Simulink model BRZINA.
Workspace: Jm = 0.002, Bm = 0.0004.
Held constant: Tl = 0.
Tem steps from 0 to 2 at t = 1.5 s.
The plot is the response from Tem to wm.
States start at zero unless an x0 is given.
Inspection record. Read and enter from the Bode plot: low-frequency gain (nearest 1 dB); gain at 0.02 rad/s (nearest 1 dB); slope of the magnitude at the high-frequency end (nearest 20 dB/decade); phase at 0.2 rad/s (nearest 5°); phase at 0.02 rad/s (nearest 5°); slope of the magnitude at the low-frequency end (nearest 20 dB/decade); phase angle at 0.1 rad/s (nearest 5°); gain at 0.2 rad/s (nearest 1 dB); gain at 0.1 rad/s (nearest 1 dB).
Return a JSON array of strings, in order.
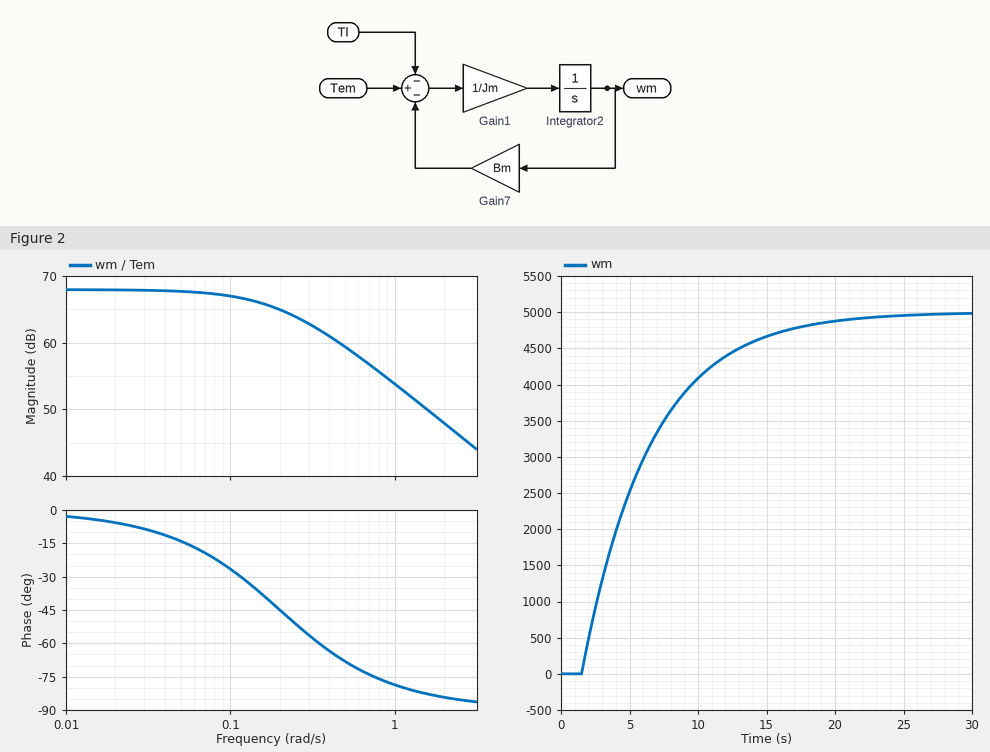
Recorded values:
["68 dB", "68 dB", "-20 dB/decade", "-45°", "-5°", "0 dB/decade", "-25°", "65 dB", "67 dB"]
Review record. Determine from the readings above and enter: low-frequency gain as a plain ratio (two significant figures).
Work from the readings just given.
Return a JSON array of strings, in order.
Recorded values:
["2500"]
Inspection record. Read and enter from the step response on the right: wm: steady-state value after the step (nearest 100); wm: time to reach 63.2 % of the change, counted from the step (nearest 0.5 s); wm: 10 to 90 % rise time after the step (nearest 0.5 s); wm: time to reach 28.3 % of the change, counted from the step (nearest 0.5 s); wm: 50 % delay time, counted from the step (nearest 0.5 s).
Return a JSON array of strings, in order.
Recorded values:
["5000", "5.0 s", "11.0 s", "1.5 s", "3.5 s"]
